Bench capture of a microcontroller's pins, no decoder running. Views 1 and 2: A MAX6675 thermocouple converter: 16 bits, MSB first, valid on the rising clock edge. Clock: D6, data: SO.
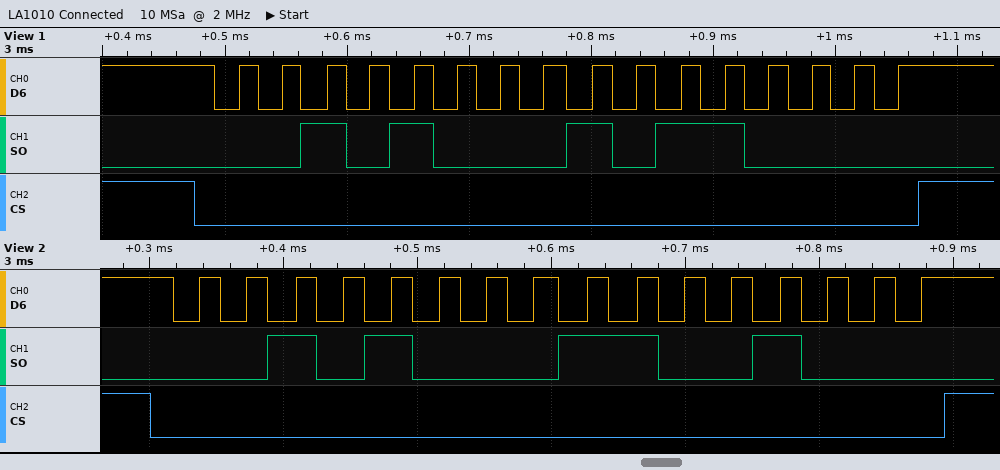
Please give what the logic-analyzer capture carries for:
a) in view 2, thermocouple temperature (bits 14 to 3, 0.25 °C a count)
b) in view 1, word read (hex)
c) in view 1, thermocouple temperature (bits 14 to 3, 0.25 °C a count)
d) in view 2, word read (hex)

326.25 °C
0x28B0
325.50 °C
0x28C8
